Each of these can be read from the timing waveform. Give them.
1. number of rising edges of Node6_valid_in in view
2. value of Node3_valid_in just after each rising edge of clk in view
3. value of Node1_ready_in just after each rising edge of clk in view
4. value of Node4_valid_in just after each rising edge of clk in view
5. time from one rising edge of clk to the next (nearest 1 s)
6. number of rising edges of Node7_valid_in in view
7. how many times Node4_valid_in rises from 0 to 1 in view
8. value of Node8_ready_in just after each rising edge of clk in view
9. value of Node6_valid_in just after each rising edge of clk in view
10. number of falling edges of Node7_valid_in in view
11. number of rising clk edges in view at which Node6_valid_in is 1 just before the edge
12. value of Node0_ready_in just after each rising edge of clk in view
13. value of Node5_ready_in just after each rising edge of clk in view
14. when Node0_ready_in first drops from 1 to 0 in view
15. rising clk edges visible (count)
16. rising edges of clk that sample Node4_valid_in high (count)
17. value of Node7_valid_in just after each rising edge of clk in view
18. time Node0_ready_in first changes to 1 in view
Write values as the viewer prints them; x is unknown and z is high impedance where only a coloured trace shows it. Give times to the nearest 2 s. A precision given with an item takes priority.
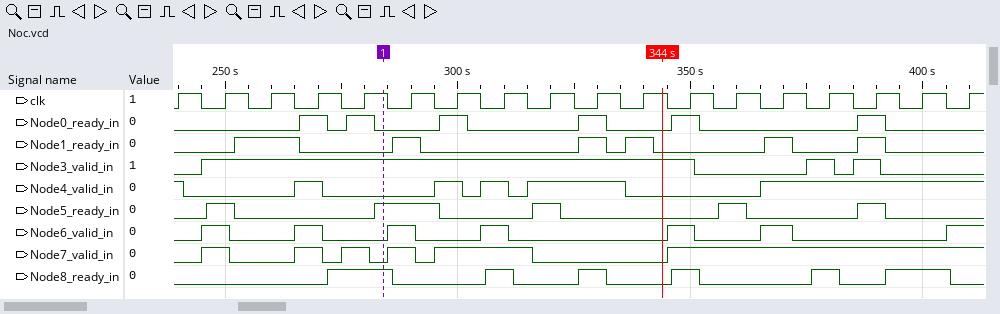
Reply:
7
0 1 1 1 1 1 1 1 1 1 1 1 0 0 1 1 0 0
0 0 1 0 0 1 0 0 0 1 1 0 0 1 0 1 0 0
1 0 0 1 0 0 1 1 1 1 0 0 0 1 1 1 1 1
10 s
6
5
0 0 0 0 1 0 0 1 0 1 0 1 0 0 1 0 1 0
0 1 0 1 0 1 0 1 0 0 0 1 0 1 0 0 0 1
5
7
0 0 0 1 1 0 1 0 0 1 0 1 0 0 0 1 0 0
0 1 0 0 0 1 0 0 1 0 0 0 1 0 0 1 0 0
272 s
18
11
0 1 0 1 1 1 1 1 0 0 0 1 1 1 1 1 1 1
266 s
